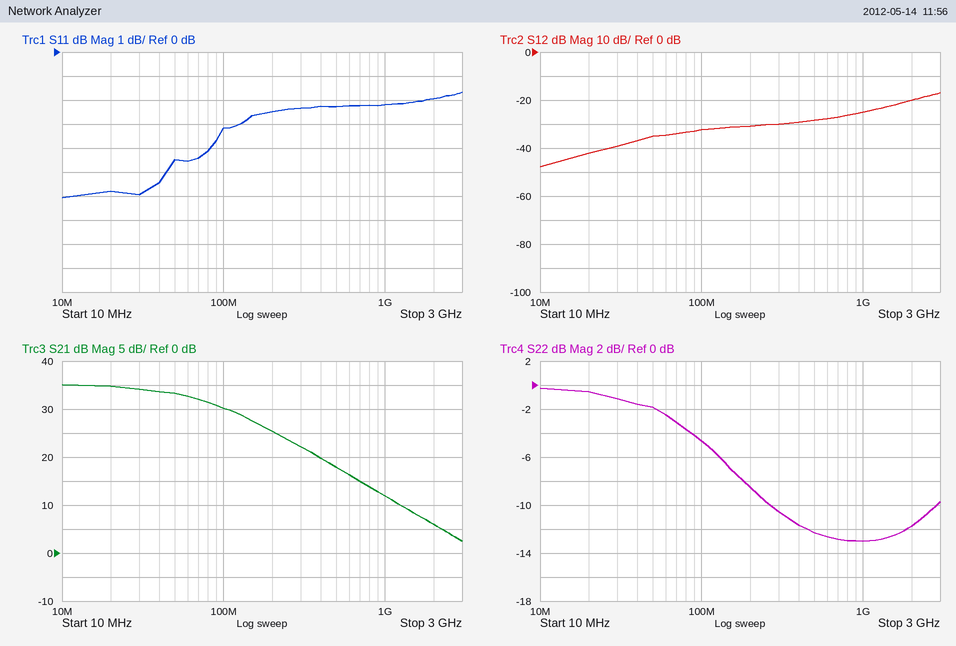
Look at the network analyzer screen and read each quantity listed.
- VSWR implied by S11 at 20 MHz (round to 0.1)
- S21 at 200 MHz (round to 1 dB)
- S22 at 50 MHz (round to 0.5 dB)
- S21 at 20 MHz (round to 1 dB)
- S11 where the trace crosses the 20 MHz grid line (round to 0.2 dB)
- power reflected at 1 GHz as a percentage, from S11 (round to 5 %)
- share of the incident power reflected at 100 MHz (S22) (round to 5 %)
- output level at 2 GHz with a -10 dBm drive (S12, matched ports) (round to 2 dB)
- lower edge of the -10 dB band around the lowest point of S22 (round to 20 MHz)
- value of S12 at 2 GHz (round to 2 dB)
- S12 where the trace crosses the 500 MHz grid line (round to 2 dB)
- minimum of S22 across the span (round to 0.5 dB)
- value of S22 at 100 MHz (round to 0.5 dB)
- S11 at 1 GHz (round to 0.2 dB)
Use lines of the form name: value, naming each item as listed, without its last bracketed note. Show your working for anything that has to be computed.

VSWR implied by S11 at 20 MHz: |Γ| = 10^(-5.8/20) = 0.5129; VSWR = (1 + 0.5129)/(1 − 0.5129) ≈ 3.1
S21 at 200 MHz: 25 dB
S22 at 50 MHz: -2.0 dB
S21 at 20 MHz: 35 dB
S11 where the trace crosses the 20 MHz grid line: -5.8 dB
power reflected at 1 GHz as a percentage, from S11: 10^(-2.2/10) ≈ 60 %
share of the incident power reflected at 100 MHz (S22): 10^(-4.5/10) ≈ 35 %
output level at 2 GHz with a -10 dBm drive (S12, matched ports): -10 dBm + (-20 dB) = -30 dBm
lower edge of the -10 dB band around the lowest point of S22: 260 MHz
value of S12 at 2 GHz: -20 dB
S12 where the trace crosses the 500 MHz grid line: -28 dB
minimum of S22 across the span: -13.0 dB
value of S22 at 100 MHz: -4.5 dB
S11 at 1 GHz: -2.2 dB
